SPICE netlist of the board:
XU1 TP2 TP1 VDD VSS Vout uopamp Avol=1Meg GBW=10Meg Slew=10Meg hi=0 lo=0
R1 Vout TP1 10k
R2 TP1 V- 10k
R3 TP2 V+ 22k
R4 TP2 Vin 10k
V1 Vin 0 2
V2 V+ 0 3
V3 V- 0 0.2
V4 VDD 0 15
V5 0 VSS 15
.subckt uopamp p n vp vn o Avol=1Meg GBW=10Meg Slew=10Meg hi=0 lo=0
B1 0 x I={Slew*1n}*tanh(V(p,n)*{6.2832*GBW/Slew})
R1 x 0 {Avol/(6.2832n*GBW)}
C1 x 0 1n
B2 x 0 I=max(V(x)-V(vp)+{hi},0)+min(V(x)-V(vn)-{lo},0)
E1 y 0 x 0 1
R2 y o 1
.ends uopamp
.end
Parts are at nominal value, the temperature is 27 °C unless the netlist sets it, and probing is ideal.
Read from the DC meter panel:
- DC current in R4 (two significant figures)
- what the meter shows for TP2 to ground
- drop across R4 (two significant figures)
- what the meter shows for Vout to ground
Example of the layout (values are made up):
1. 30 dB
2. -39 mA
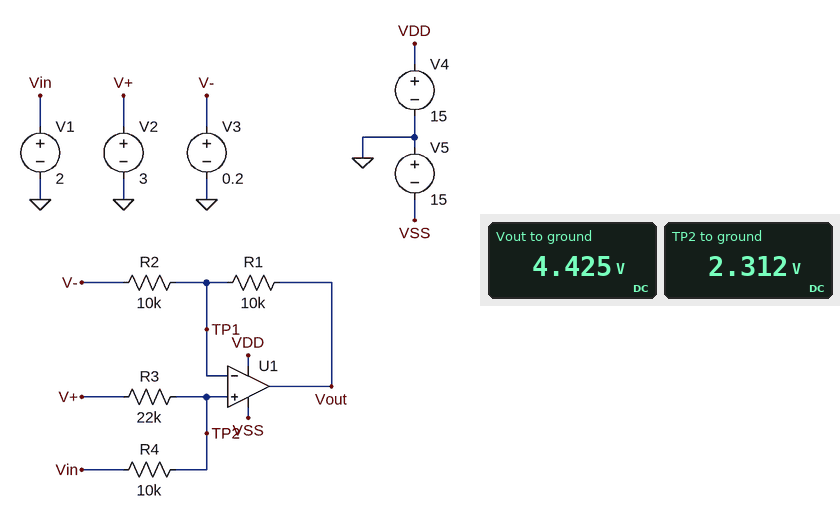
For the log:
1. 31 µA
2. 2.312 V
3. 310 mV
4. 4.425 V
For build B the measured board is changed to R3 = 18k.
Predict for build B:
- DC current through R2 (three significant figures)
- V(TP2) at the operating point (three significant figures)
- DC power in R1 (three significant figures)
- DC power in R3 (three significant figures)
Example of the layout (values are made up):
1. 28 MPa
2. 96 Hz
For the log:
1. 216 µA
2. 2.36 V
3. 465 µW
4. 23.0 µW
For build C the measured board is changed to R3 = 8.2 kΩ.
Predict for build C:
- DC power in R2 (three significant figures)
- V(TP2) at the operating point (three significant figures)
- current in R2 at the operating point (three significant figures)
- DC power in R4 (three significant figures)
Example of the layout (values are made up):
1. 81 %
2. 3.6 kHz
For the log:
1. 552 µW
2. 2.55 V
3. 235 µA
4. 30.2 µW
